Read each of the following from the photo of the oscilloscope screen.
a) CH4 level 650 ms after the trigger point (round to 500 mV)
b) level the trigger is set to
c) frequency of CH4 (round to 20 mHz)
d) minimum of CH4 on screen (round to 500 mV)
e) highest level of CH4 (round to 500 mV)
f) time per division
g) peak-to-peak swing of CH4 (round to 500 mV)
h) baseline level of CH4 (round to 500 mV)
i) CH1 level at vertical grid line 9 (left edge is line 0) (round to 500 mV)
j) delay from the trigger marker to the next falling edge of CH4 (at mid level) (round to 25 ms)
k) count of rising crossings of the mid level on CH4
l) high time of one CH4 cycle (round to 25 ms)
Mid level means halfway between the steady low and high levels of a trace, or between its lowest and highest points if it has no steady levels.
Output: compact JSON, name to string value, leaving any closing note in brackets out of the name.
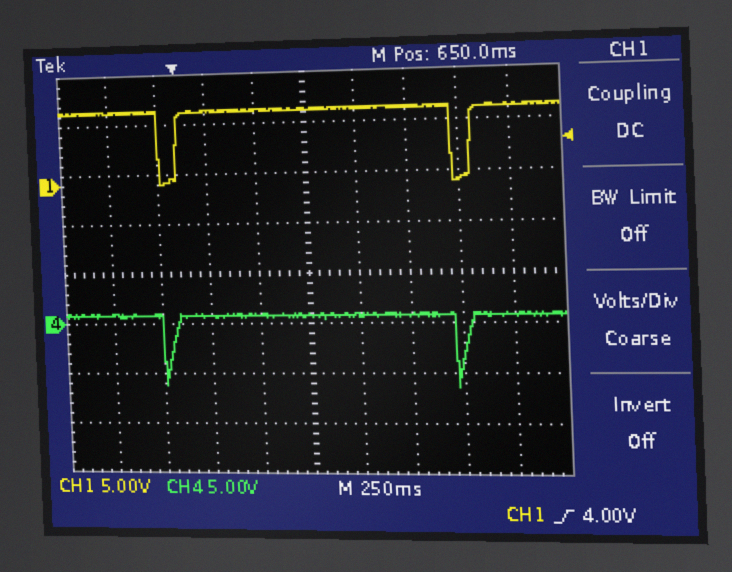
{"CH4 level 650 ms after the trigger point": "1.0 V", "level the trigger is set to": "4.00 V", "frequency of CH4": "680 mHz", "minimum of CH4 on screen": "-6.5 V", "highest level of CH4": "1.0 V", "time per division": "250 ms", "peak-to-peak swing of CH4": "7.5 V", "baseline level of CH4": "1.0 V", "CH1 level at vertical grid line 9 (left edge is line 0)": "7.5 V", "delay from the trigger marker to the next falling edge of CH4 (at mid level)": "1.375 s", "count of rising crossings of the mid level on CH4": "2", "high time of one CH4 cycle": "1.425 s"}
